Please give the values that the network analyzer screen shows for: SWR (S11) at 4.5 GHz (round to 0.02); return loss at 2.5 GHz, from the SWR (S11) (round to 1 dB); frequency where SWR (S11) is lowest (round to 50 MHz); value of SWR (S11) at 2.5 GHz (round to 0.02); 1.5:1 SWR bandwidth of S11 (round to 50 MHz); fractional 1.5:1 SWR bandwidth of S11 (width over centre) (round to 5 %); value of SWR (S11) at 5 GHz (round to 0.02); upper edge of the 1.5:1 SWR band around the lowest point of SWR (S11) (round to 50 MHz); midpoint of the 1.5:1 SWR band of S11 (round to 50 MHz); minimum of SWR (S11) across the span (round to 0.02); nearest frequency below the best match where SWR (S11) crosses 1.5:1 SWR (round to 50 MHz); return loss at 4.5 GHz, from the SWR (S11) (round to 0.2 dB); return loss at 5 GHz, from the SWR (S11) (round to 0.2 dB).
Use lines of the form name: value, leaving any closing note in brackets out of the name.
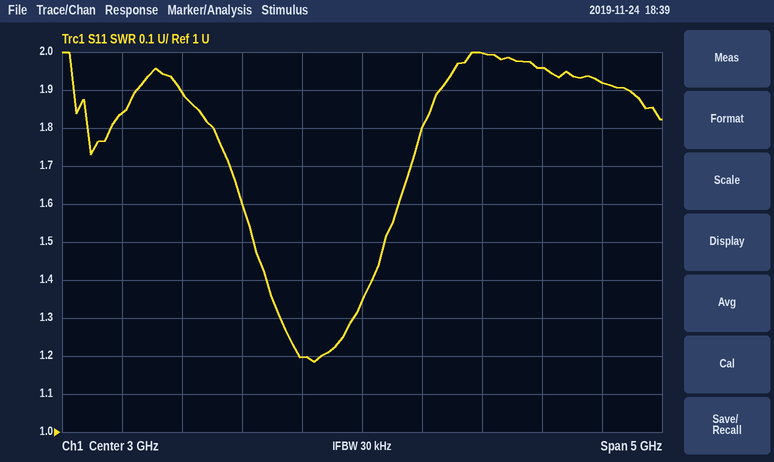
SWR (S11) at 4.5 GHz: 1.96
return loss at 2.5 GHz, from the SWR (S11): 21 dB
frequency where SWR (S11) is lowest: 2.60 GHz
value of SWR (S11) at 2.5 GHz: 1.20
1.5:1 SWR bandwidth of S11: 1.10 GHz
fractional 1.5:1 SWR bandwidth of S11 (width over centre): 40 %
value of SWR (S11) at 5 GHz: 1.92
upper edge of the 1.5:1 SWR band around the lowest point of SWR (S11): 3.20 GHz
midpoint of the 1.5:1 SWR band of S11: 2.65 GHz
minimum of SWR (S11) across the span: 1.18
nearest frequency below the best match where SWR (S11) crosses 1.5:1 SWR: 2.10 GHz
return loss at 4.5 GHz, from the SWR (S11): 9.8 dB
return loss at 5 GHz, from the SWR (S11): 10.0 dB
